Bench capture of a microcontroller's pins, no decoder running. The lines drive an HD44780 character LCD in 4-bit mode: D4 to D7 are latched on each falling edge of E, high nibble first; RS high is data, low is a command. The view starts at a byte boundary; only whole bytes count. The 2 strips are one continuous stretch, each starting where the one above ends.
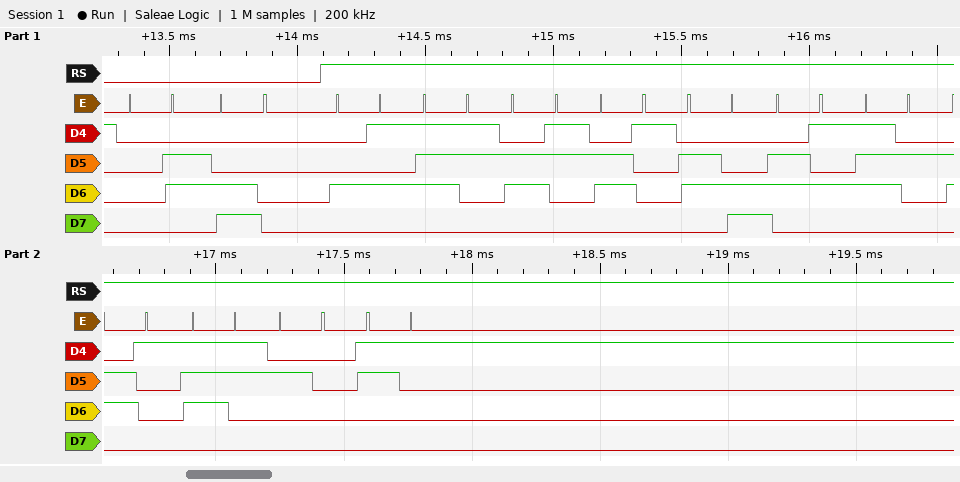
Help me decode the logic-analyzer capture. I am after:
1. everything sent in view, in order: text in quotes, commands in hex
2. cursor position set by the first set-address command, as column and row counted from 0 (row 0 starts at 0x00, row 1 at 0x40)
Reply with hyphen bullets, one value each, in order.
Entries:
- 0x06 0xC0 "Escaleras 1"
- column 0, row 1
